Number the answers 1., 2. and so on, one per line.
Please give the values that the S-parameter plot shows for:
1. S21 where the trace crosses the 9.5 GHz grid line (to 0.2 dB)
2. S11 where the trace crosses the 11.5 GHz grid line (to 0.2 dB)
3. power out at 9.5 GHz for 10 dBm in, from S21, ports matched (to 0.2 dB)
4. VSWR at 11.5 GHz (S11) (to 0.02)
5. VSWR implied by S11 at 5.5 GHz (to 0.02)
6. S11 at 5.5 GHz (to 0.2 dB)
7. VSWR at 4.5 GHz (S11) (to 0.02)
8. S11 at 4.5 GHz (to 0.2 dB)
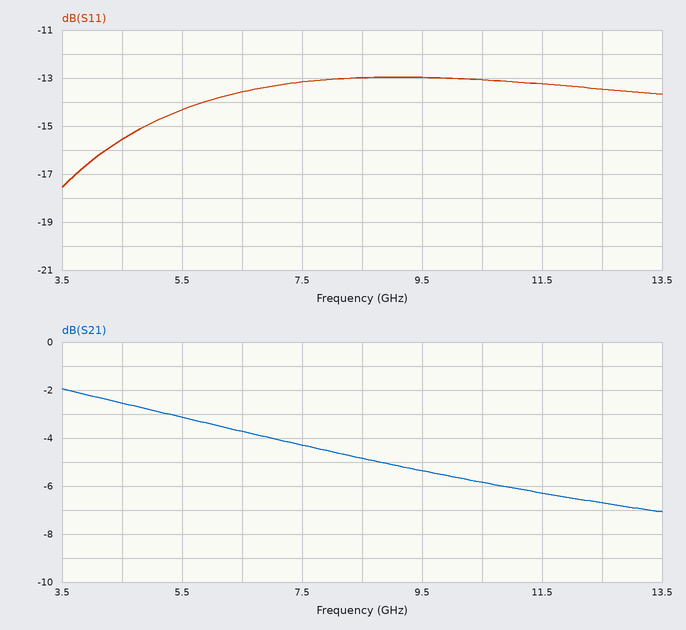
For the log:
1. -5.4 dB
2. -13.2 dB
3. 4.6 dBm
4. 1.56
5. 1.48
6. -14.4 dB
7. 1.40
8. -15.6 dB
